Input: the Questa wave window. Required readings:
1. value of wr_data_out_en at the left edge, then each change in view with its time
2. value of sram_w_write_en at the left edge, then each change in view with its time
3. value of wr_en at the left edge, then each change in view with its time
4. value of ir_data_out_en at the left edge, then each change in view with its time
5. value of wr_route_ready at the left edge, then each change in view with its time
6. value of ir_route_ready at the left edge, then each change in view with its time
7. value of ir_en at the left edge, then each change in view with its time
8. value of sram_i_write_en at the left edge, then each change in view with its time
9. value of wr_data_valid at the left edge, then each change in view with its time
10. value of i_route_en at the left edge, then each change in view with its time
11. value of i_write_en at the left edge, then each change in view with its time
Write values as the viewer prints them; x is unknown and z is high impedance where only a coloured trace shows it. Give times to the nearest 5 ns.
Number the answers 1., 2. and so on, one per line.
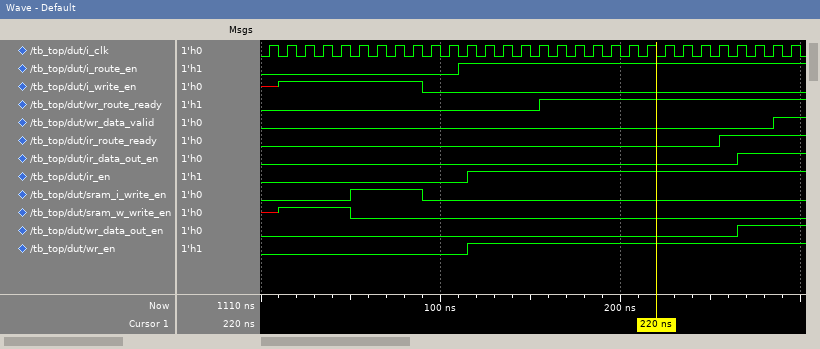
1. 0, 1 at 265 ns
2. x, 1 at 10 ns, 0 at 50 ns
3. 0, 1 at 115 ns
4. 0, 1 at 265 ns
5. 0, 1 at 155 ns
6. 0, 1 at 255 ns
7. 0, 1 at 115 ns
8. 0, 1 at 50 ns, 0 at 90 ns
9. 0, 1 at 285 ns
10. 0, 1 at 110 ns
11. x, 1 at 10 ns, 0 at 90 ns
